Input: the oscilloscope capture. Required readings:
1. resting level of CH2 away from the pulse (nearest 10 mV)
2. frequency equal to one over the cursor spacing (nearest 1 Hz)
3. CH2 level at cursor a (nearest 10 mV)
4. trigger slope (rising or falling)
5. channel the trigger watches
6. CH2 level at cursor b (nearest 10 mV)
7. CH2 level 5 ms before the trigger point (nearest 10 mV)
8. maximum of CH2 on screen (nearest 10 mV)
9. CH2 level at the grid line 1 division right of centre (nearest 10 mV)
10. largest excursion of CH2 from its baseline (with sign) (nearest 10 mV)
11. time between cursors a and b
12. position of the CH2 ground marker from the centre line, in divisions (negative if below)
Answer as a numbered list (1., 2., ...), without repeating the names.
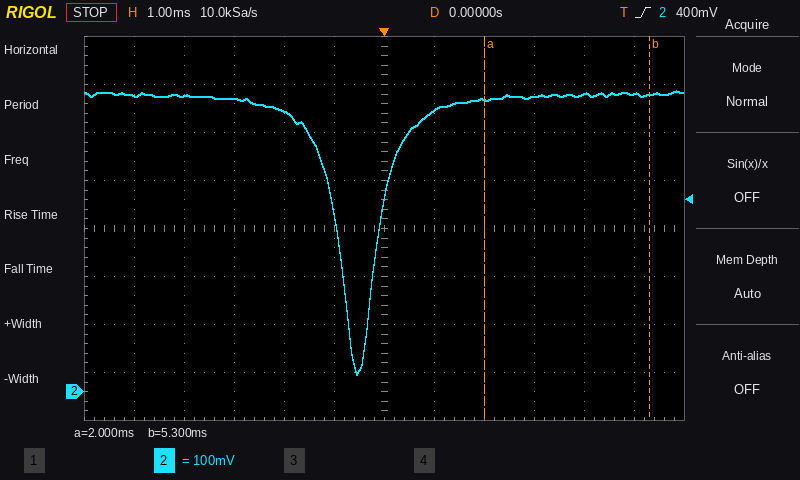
1. 620 mV
2. 303 Hz
3. 610 mV
4. rising
5. CH2
6. 620 mV
7. 620 mV
8. 630 mV
9. 590 mV
10. -580 mV
11. 3.3 ms
12. -3.4 div
